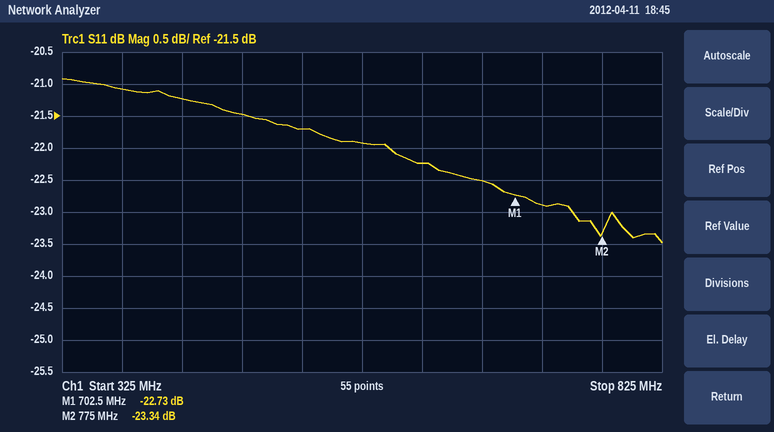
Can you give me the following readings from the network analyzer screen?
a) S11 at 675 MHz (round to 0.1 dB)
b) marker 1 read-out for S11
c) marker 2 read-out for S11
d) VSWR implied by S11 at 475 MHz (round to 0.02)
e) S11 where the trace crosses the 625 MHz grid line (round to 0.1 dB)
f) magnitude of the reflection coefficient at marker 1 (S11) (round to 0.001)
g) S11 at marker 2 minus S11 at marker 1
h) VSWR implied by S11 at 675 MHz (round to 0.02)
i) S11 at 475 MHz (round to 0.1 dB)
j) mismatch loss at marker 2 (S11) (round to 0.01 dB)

-22.5 dB
-22.73 dB
-23.34 dB
1.18
-22.2 dB
0.073
-0.61 dB
1.16
-21.5 dB
0.02 dB
